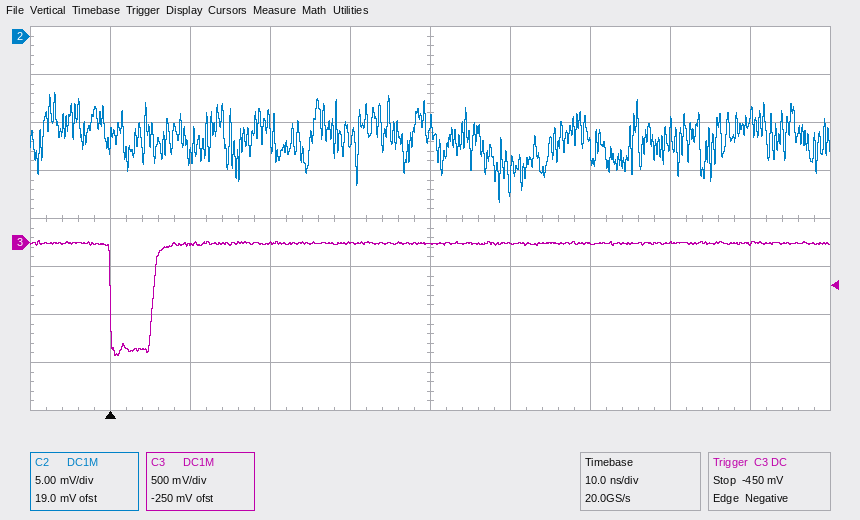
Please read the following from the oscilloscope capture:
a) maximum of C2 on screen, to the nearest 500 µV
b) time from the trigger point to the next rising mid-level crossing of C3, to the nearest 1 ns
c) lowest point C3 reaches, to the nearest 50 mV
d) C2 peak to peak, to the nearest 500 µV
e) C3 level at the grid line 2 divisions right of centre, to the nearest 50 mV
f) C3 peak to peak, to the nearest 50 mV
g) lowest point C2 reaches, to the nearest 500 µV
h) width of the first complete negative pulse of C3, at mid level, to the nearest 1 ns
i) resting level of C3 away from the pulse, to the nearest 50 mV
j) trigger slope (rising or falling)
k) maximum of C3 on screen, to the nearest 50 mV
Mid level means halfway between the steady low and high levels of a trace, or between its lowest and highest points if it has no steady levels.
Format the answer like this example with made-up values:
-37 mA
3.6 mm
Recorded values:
-6.0 mV
5 ns
-1.20 V
11.5 mV
0 mV
1.20 V
-17.5 mV
5 ns
0 mV
falling
0 mV
